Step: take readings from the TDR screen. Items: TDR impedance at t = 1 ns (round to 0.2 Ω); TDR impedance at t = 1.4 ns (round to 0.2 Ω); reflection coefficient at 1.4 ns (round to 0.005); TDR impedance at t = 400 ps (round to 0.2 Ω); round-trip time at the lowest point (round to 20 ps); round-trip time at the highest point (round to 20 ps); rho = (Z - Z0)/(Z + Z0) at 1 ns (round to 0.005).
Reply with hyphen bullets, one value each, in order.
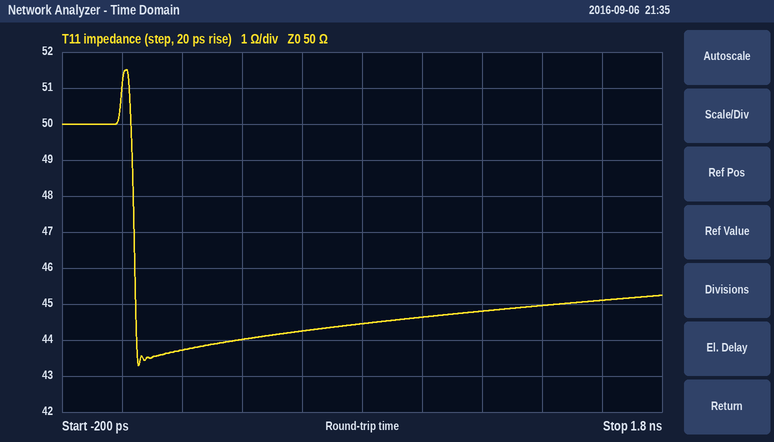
- 44.6 Ω
- 45.0 Ω
- -0.055
- 44.0 Ω
- 60 ps
- 20 ps
- -0.055
